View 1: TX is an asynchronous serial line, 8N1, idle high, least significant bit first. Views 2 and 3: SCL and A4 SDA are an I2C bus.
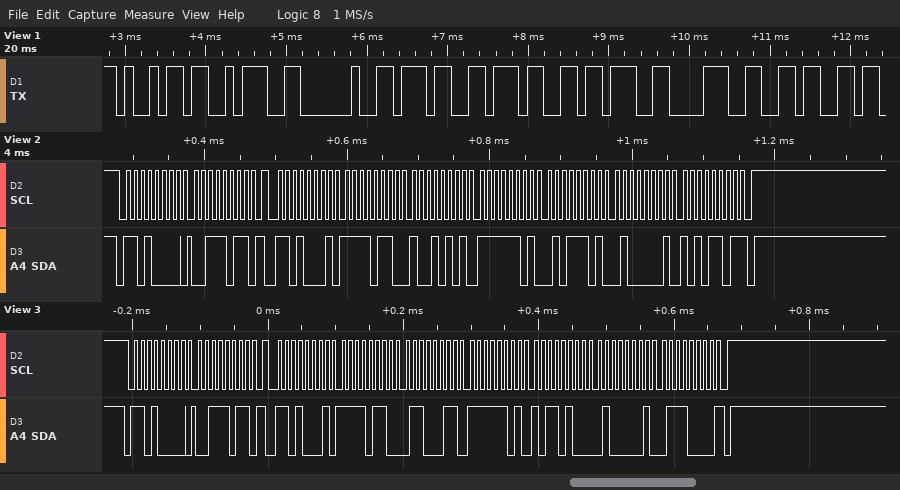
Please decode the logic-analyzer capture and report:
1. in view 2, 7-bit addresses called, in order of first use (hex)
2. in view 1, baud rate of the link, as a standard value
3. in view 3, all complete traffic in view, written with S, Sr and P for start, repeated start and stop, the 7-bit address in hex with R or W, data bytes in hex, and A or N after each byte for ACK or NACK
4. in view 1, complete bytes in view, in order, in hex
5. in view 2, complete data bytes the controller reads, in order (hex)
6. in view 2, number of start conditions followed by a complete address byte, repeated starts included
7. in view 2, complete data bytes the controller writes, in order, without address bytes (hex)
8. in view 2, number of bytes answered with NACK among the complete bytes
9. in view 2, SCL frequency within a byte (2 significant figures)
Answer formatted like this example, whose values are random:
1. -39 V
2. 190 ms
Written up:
1. 0x68
2. 9600 baud
3. S 68W A 3B A Sr 68R A F6 A 63 A FD A B4 A 41 A 70 N P
4. 69 3A 20 37 37 3B 38 36
5. F6 95 FD 5D 41 AD
6. 2
7. 3B
8. 1
9. 100 kHz
